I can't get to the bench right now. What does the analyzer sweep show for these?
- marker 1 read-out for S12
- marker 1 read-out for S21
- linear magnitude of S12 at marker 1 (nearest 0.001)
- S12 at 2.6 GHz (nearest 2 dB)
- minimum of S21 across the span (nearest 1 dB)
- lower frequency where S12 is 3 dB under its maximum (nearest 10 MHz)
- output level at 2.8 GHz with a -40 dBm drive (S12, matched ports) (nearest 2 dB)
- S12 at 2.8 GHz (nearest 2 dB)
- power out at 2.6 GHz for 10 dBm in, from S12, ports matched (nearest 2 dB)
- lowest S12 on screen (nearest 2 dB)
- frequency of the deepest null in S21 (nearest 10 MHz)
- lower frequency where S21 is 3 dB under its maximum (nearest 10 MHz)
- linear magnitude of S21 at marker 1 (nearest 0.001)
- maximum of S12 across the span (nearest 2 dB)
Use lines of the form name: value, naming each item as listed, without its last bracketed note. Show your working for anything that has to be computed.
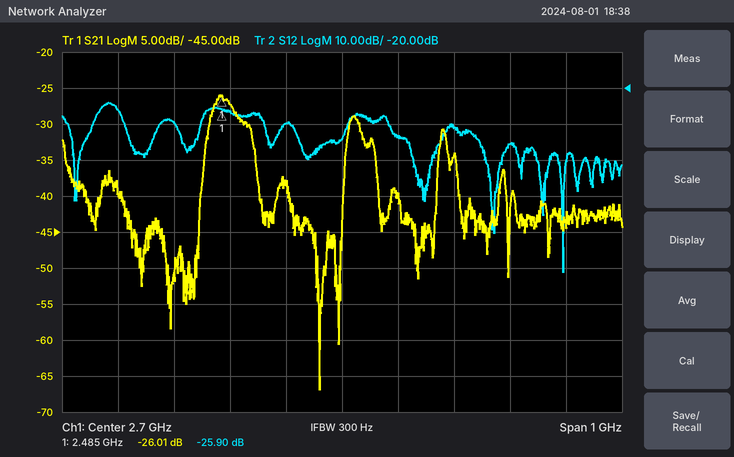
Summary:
marker 1 read-out for S12: -25.90 dB
marker 1 read-out for S21: -26.01 dB
linear magnitude of S12 at marker 1: 10^(-25.9/20) ≈ 0.051
S12 at 2.6 GHz: -30 dB
minimum of S21 across the span: -67 dB
lower frequency where S12 is 3 dB under its maximum: 2.26 GHz
output level at 2.8 GHz with a -40 dBm drive (S12, matched ports): -40 dBm + (-34 dB) = -74 dBm
S12 at 2.8 GHz: -34 dB
power out at 2.6 GHz for 10 dBm in, from S12, ports matched: 10 dBm + (-30 dB) = -20 dBm
lowest S12 on screen: -72 dB
frequency of the deepest null in S21: 2.66 GHz
lower frequency where S21 is 3 dB under its maximum: 2.47 GHz
linear magnitude of S21 at marker 1: 10^(-26.01/20) ≈ 0.050
maximum of S12 across the span: -24 dB
